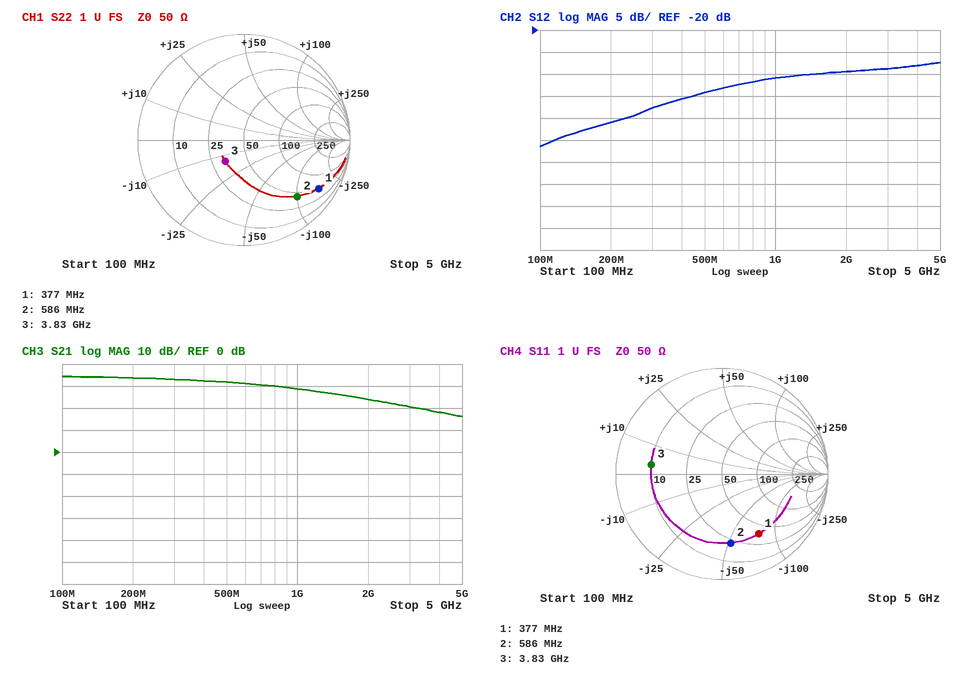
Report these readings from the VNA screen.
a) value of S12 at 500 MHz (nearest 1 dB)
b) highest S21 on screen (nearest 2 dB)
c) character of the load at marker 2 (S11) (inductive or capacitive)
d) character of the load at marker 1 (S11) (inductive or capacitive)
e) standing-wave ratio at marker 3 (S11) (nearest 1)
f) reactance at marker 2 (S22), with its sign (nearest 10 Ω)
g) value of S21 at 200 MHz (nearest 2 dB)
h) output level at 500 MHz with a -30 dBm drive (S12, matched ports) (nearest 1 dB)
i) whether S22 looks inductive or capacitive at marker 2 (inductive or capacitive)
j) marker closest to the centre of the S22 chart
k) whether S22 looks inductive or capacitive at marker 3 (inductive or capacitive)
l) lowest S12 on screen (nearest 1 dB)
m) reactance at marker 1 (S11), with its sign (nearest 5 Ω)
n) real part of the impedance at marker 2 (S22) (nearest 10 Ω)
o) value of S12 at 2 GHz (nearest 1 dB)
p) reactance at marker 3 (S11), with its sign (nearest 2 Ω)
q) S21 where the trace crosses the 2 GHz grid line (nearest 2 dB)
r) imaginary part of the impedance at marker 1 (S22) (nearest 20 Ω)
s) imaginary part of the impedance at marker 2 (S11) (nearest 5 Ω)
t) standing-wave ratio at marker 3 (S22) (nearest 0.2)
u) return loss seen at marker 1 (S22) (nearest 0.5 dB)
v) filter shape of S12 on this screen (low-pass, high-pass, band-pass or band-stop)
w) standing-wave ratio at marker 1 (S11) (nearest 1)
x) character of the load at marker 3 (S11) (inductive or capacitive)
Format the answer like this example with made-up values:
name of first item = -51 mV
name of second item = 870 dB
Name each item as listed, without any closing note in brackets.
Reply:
value of S12 at 500 MHz = -34 dB
highest S21 on screen = 34 dB
character of the load at marker 2 (S11) = capacitive
character of the load at marker 1 (S11) = capacitive
standing-wave ratio at marker 3 (S11) = 5
reactance at marker 2 (S22), with its sign = -100 Ω
value of S21 at 200 MHz = 34 dB
output level at 500 MHz with a -30 dBm drive (S12, matched ports) = -64 dBm
whether S22 looks inductive or capacitive at marker 2 = capacitive
marker closest to the centre of the S22 chart = marker 3
whether S22 looks inductive or capacitive at marker 3 = capacitive
lowest S12 on screen = -46 dB
reactance at marker 1 (S11), with its sign = -75 Ω
real part of the impedance at marker 2 (S22) = 40 Ω
value of S12 at 2 GHz = -29 dB
reactance at marker 3 (S11), with its sign = +4 Ω
S21 where the trace crosses the 2 GHz grid line = 24 dB
imaginary part of the impedance at marker 1 (S22) = -160 Ω
imaginary part of the impedance at marker 2 (S11) = -50 Ω
standing-wave ratio at marker 3 (S22) = 1.8
return loss seen at marker 1 (S22) = 1.5 dB
filter shape of S12 on this screen = high-pass
standing-wave ratio at marker 1 (S11) = 5
character of the load at marker 3 (S11) = inductive
